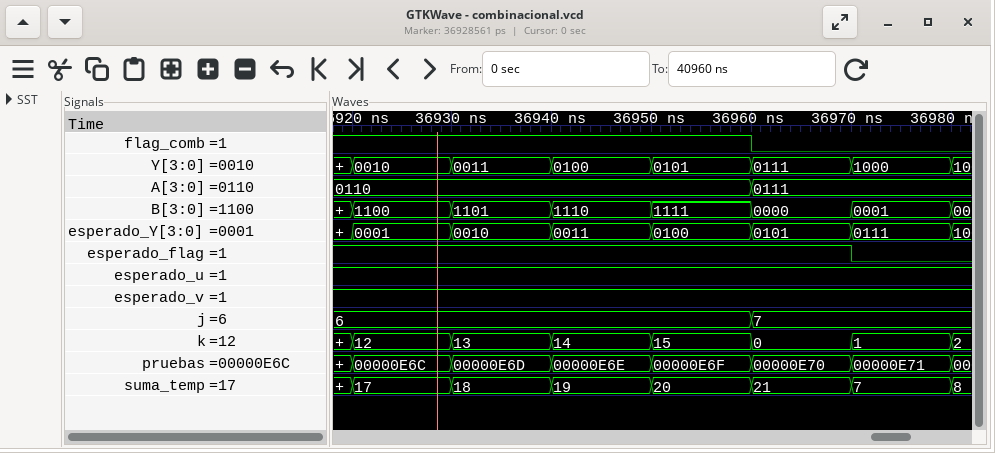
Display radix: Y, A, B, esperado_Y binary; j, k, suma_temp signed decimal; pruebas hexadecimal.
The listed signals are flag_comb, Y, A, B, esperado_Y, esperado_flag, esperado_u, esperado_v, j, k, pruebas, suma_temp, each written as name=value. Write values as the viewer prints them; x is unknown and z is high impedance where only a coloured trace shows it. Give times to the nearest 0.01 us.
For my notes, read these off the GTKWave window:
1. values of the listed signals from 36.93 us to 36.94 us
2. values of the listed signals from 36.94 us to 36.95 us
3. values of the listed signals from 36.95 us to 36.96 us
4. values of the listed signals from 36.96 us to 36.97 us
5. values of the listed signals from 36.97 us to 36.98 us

flag_comb=1, Y=0011, A=0110, B=1101, esperado_Y=0010, esperado_flag=1, esperado_u=1, esperado_v=1, j=6, k=13, pruebas=00000E6D, suma_temp=18
flag_comb=1, Y=0100, A=0110, B=1110, esperado_Y=0011, esperado_flag=1, esperado_u=1, esperado_v=1, j=6, k=14, pruebas=00000E6E, suma_temp=19
flag_comb=1, Y=0101, A=0110, B=1111, esperado_Y=0100, esperado_flag=1, esperado_u=1, esperado_v=1, j=6, k=15, pruebas=00000E6F, suma_temp=20
flag_comb=0, Y=0111, A=0111, B=0000, esperado_Y=0101, esperado_flag=1, esperado_u=1, esperado_v=1, j=7, k=0, pruebas=00000E70, suma_temp=21
flag_comb=0, Y=1000, A=0111, B=0001, esperado_Y=0111, esperado_flag=0, esperado_u=1, esperado_v=1, j=7, k=1, pruebas=00000E71, suma_temp=7
